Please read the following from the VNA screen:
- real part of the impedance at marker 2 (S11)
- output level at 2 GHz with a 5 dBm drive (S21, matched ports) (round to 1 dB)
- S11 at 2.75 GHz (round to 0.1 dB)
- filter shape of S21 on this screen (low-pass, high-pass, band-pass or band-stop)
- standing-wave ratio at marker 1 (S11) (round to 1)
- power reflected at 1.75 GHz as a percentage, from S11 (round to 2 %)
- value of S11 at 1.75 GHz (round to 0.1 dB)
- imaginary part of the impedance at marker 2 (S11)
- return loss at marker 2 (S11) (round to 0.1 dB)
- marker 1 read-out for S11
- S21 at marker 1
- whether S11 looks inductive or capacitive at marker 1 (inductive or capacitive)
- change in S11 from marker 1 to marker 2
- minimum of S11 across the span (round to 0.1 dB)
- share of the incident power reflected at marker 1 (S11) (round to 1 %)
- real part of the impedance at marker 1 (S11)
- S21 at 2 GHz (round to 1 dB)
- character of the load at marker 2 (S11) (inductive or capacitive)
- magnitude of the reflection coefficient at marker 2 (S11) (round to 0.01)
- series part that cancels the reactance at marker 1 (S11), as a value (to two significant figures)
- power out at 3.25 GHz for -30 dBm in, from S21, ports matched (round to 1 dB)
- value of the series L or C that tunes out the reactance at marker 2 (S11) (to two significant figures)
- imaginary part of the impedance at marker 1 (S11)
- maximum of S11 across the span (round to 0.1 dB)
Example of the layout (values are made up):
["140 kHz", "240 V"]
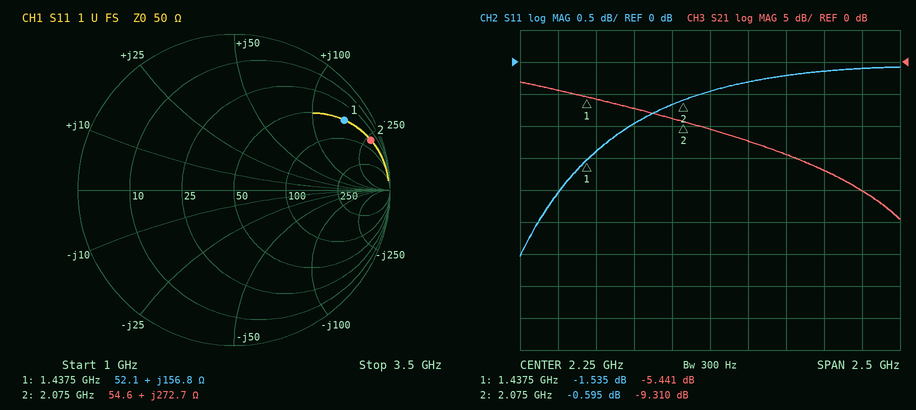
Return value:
["54.6 Ω", "-4 dBm", "-0.2 dB", "low-pass", "11", "80 %", "-1.0 dB", "+272.7 Ω", "0.6 dB", "-1.535 dB", "-5.441 dB", "inductive", "0.940 dB", "-3.0 dB", "70 %", "52.1 Ω", "-9 dB", "inductive", "0.93", "710 fF", "-50 dBm", "280 fF", "+156.8 Ω", "-0.1 dB"]
